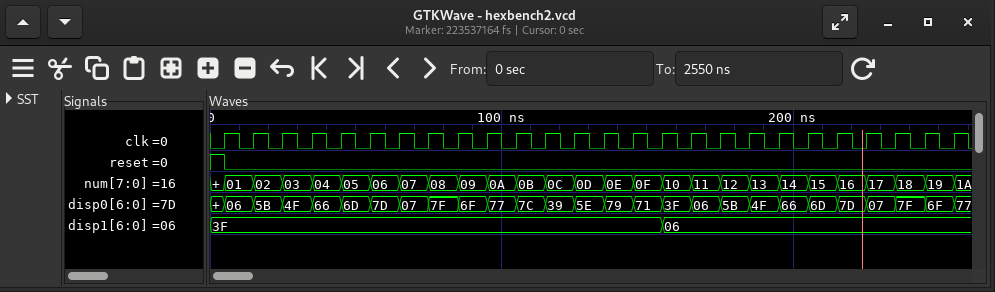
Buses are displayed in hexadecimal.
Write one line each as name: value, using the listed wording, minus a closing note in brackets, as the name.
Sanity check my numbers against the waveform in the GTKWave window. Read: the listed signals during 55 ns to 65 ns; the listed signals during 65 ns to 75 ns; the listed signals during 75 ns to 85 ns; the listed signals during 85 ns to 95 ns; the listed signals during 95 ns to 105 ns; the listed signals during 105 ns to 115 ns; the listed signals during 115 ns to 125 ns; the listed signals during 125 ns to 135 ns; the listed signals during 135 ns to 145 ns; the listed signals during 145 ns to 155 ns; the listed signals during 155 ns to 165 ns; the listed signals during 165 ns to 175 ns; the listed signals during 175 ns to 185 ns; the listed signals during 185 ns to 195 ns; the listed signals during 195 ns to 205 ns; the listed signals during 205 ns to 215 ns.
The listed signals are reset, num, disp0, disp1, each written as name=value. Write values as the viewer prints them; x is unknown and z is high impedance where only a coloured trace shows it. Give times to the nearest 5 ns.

the listed signals during 55 ns to 65 ns: reset=0, num=06, disp0=7D, disp1=3F
the listed signals during 65 ns to 75 ns: reset=0, num=07, disp0=07, disp1=3F
the listed signals during 75 ns to 85 ns: reset=0, num=08, disp0=7F, disp1=3F
the listed signals during 85 ns to 95 ns: reset=0, num=09, disp0=6F, disp1=3F
the listed signals during 95 ns to 105 ns: reset=0, num=0A, disp0=77, disp1=3F
the listed signals during 105 ns to 115 ns: reset=0, num=0B, disp0=7C, disp1=3F
the listed signals during 115 ns to 125 ns: reset=0, num=0C, disp0=39, disp1=3F
the listed signals during 125 ns to 135 ns: reset=0, num=0D, disp0=5E, disp1=3F
the listed signals during 135 ns to 145 ns: reset=0, num=0E, disp0=79, disp1=3F
the listed signals during 145 ns to 155 ns: reset=0, num=0F, disp0=71, disp1=3F
the listed signals during 155 ns to 165 ns: reset=0, num=10, disp0=3F, disp1=06
the listed signals during 165 ns to 175 ns: reset=0, num=11, disp0=06, disp1=06
the listed signals during 175 ns to 185 ns: reset=0, num=12, disp0=5B, disp1=06
the listed signals during 185 ns to 195 ns: reset=0, num=13, disp0=4F, disp1=06
the listed signals during 195 ns to 205 ns: reset=0, num=14, disp0=66, disp1=06
the listed signals during 205 ns to 215 ns: reset=0, num=15, disp0=6D, disp1=06
